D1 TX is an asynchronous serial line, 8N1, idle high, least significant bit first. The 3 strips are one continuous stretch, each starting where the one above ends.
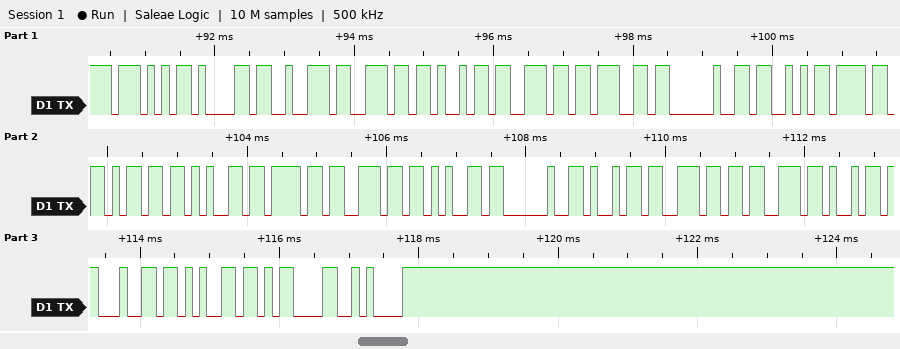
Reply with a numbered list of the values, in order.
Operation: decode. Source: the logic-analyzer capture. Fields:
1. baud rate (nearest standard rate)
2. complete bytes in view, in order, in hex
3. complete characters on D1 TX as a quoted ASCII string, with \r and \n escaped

1. 9600 baud
2. 57 61 72 6E 69 6E 67 20 53 6F 6D 65 6F 6E 65 20 69 6E 73 69 64 65 0D 0A
3. "Warning Someone inside\r\n"
